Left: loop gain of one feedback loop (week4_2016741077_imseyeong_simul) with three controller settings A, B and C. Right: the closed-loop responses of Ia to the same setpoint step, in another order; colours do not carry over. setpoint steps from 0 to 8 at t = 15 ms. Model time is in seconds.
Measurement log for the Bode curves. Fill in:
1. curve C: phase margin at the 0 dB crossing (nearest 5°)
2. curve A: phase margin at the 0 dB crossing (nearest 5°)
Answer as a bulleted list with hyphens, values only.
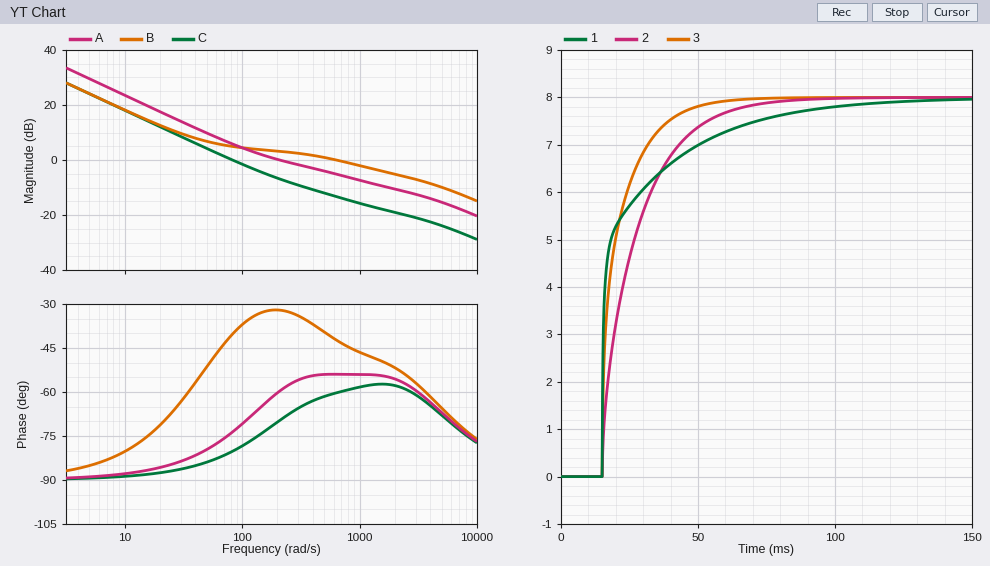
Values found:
- 100°
- 120°
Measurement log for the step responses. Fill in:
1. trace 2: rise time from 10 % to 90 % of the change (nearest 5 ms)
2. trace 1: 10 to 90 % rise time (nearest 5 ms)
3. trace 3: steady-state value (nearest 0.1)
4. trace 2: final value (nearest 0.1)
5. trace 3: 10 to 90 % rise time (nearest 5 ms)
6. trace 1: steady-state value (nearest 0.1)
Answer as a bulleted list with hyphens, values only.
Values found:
- 30 ms
- 40 ms
- 8.0
- 8.0
- 20 ms
- 8.0
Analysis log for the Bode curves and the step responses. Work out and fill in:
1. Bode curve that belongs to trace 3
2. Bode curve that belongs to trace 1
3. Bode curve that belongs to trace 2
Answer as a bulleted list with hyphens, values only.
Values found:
- A
- B
- C
